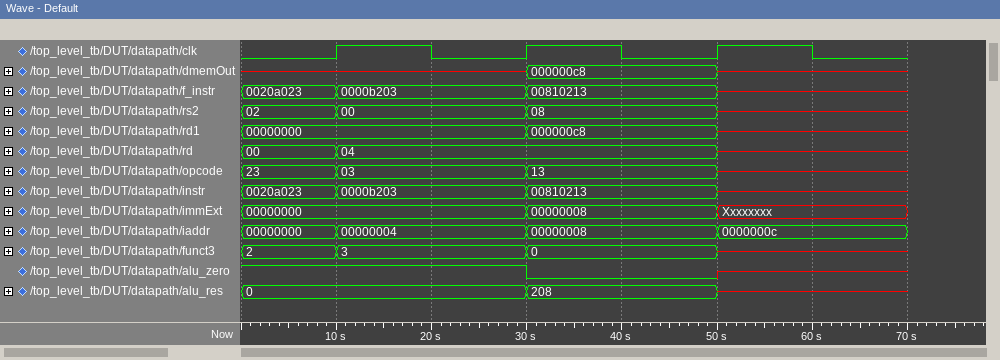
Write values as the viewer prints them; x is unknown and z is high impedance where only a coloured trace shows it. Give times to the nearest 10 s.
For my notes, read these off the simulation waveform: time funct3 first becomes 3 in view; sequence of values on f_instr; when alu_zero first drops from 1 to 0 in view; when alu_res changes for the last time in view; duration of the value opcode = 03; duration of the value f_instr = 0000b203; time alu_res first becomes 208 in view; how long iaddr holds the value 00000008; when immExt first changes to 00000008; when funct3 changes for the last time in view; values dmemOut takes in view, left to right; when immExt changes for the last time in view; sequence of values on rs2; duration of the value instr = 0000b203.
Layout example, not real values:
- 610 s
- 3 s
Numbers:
- 10 s
- 0020a023, 0000b203, 00810213, x
- 30 s
- 50 s
- 20 s
- 20 s
- 30 s
- 20 s
- 30 s
- 50 s
- x, 000000c8, x
- 50 s
- 02, 00, 08, x
- 20 s
